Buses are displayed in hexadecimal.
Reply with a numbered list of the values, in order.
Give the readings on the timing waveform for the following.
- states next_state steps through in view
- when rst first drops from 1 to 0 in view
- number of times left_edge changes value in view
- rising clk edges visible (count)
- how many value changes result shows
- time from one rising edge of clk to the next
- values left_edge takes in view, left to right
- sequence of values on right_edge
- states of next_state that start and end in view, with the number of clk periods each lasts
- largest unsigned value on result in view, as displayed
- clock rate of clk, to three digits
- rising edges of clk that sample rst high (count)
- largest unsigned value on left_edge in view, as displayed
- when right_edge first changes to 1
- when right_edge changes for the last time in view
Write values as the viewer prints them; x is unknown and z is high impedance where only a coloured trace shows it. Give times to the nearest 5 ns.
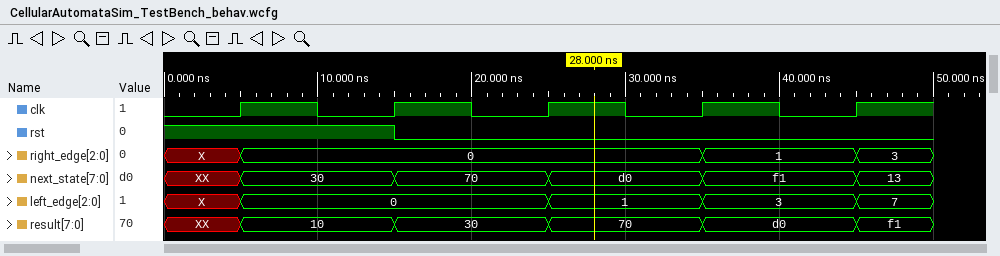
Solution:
1. XX, 30, 70, d0, f1, 13
2. 15 ns
3. 4
4. 5
5. 5
6. 10 ns
7. X, 0, 1, 3, 7
8. X, 0, 1, 3
9. 30: 1, 70: 1, d0: 1, f1: 1
10. f1
11. 100 MHz
12. 2
13. 7
14. 35 ns
15. 45 ns
